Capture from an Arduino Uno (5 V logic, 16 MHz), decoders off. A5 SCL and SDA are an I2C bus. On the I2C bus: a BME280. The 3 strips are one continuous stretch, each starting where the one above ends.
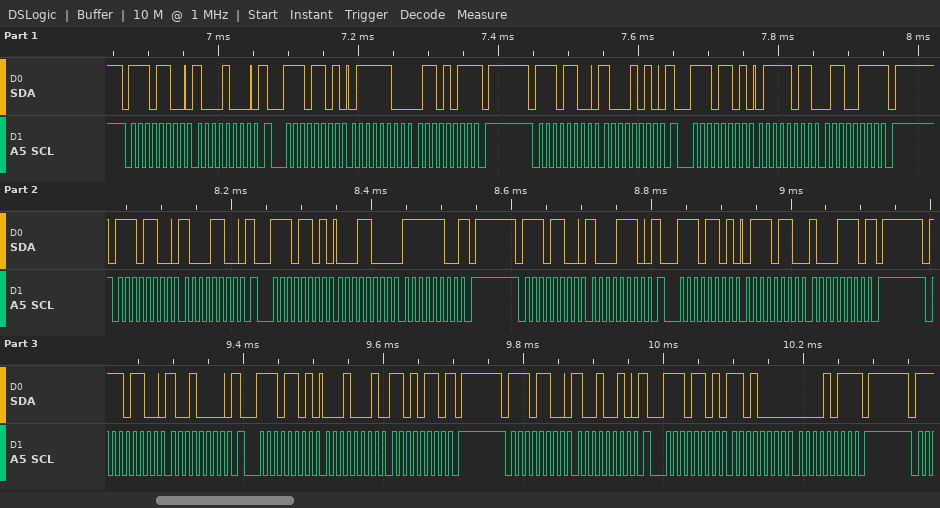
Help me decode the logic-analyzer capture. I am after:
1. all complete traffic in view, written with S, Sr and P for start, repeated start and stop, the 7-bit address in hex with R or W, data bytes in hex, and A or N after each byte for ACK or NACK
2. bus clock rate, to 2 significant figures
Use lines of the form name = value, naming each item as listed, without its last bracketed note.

all complete traffic in view, written with S, Sr and P for start, repeated start and stop, the 7-bit address in hex with R or W, data bytes in hex, and A or N after each byte for ACK or NACK = S 76W A 88 A Sr 76R A 7C A 6B N P S 76W A 8A A Sr 76R A 7B A 67 N P S 76W A 8C A Sr 76R A 18 A FC N P S 76W A 8E A Sr 76R A 76 A 8E N P S 76W A 90 A Sr 76R A 11 A D6 N P S 76W A 92 A Sr 76R A D0 A 0B N P
bus clock rate, to 2 significant figures = 100 kHz
